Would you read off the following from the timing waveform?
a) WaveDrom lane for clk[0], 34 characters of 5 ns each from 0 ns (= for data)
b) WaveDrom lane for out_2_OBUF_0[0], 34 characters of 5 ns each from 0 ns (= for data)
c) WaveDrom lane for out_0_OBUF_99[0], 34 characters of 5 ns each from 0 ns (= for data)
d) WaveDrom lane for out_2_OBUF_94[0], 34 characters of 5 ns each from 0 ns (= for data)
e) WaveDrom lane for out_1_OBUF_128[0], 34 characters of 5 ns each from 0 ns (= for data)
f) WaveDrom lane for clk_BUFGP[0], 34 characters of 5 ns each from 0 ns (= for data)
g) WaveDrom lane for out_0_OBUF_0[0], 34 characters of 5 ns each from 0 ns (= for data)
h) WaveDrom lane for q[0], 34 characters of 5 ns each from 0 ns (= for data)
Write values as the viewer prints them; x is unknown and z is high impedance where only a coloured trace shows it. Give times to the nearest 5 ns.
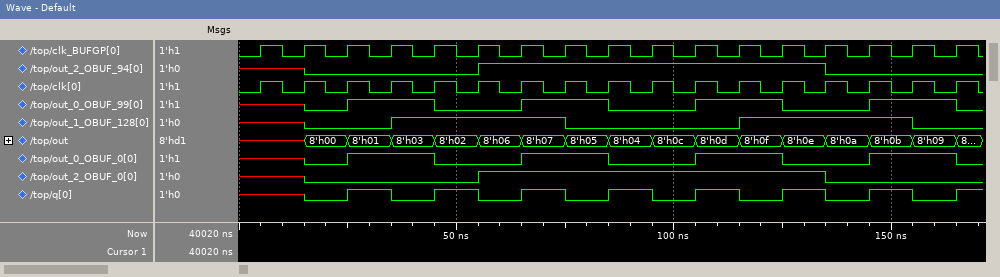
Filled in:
{name: 'clk[0]', wave: '0101010101010101010101010101010101'}
{name: 'out_2_OBUF_0[0]', wave: 'x..0.......1...............0......'}
{name: 'out_0_OBUF_99[0]', wave: 'x..0.1...0...1...0...1...0...1...0'}
{name: 'out_2_OBUF_94[0]', wave: 'x..0.......1...............0......'}
{name: 'out_1_OBUF_128[0]', wave: 'x..0...1.......0.......1.......0..'}
{name: 'clk_BUFGP[0]', wave: '0101010101010101010101010101010101'}
{name: 'out_0_OBUF_0[0]', wave: 'x..0.1...0...1...0...1...0...1...0'}
{name: 'q[0]', wave: 'x..0.1.0.1.0.1.0.1.0.1.0.1.0.1.0.1'}
